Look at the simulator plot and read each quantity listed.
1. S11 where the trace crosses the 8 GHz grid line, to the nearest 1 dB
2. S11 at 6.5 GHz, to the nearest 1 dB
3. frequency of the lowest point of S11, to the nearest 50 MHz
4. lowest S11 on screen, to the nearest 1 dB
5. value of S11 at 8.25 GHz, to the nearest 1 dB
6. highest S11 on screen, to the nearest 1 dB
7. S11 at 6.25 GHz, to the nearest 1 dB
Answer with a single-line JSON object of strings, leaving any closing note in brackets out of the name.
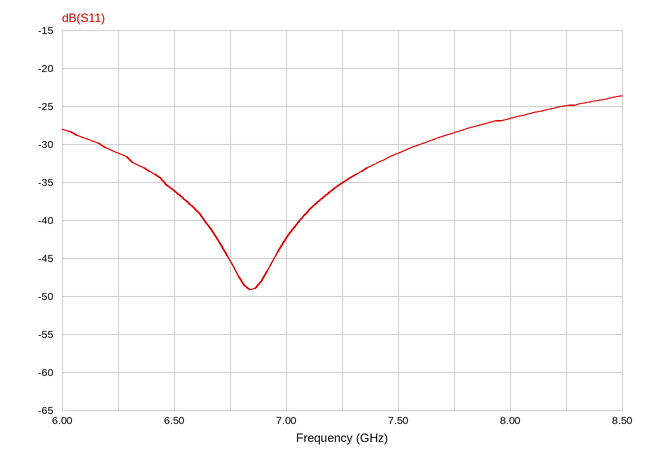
{"S11 where the trace crosses the 8 GHz grid line, to the nearest 1 dB": "-27 dB", "S11 at 6.5 GHz, to the nearest 1 dB": "-36 dB", "frequency of the lowest point of S11, to the nearest 50 MHz": "6.85 GHz", "lowest S11 on screen, to the nearest 1 dB": "-49 dB", "value of S11 at 8.25 GHz, to the nearest 1 dB": "-25 dB", "highest S11 on screen, to the nearest 1 dB": "-24 dB", "S11 at 6.25 GHz, to the nearest 1 dB": "-31 dB"}
